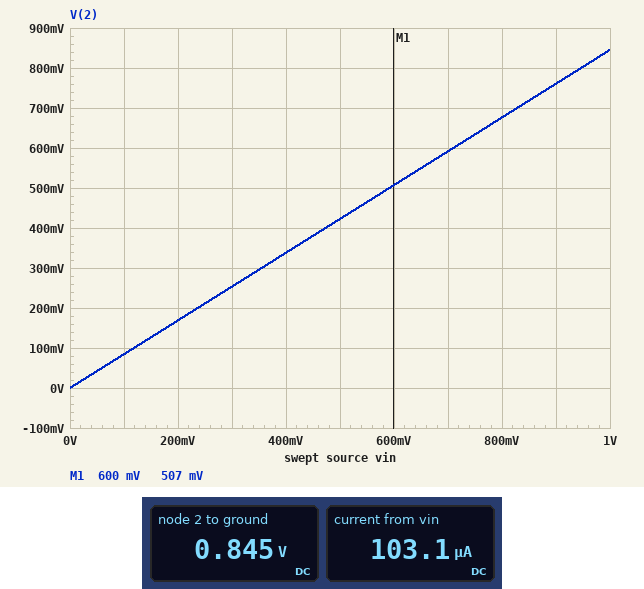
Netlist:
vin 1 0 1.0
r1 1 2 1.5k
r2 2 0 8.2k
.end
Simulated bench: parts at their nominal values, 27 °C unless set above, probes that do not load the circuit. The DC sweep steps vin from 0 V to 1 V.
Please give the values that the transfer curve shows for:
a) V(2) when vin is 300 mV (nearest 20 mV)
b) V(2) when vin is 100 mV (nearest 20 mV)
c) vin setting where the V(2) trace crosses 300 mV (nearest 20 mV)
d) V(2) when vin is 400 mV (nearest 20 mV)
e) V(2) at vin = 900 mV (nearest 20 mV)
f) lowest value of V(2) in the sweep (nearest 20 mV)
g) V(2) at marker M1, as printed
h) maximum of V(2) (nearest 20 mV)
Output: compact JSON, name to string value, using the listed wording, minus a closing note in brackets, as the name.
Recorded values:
{"V(2) when vin is 300 mV": "260 mV", "V(2) when vin is 100 mV": "80 mV", "vin setting where the V(2) trace crosses 300 mV": "360 mV", "V(2) when vin is 400 mV": "340 mV", "V(2) at vin = 900 mV": "760 mV", "lowest value of V(2) in the sweep": "0 V", "V(2) at marker M1, as printed": "507 mV", "maximum of V(2)": "840 mV"}
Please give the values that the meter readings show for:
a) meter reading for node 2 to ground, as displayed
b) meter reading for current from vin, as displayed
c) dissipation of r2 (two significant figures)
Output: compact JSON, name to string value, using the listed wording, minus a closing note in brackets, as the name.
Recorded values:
{"meter reading for node 2 to ground, as displayed": "0.845 V", "meter reading for current from vin, as displayed": "103.1 µA", "dissipation of r2": "87 µW"}
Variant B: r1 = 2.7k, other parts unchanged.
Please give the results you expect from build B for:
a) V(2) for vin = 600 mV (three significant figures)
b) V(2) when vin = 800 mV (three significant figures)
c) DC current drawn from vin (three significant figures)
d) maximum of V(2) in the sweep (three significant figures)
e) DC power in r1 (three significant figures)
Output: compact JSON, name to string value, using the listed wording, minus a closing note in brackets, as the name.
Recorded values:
{"V(2) for vin = 600 mV": "451 mV", "V(2) when vin = 800 mV": "602 mV", "DC current drawn from vin": "91.7 µA", "maximum of V(2) in the sweep": "752 mV", "DC power in r1": "22.7 µW"}
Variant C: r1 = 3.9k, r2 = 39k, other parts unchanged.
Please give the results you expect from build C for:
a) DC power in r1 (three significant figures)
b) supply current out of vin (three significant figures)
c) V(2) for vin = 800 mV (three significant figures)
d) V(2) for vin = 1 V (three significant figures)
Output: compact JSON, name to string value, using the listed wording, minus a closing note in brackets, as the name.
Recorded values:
{"DC power in r1": "2.12 µW", "supply current out of vin": "23.3 µA", "V(2) for vin = 800 mV": "727 mV", "V(2) for vin = 1 V": "909 mV"}
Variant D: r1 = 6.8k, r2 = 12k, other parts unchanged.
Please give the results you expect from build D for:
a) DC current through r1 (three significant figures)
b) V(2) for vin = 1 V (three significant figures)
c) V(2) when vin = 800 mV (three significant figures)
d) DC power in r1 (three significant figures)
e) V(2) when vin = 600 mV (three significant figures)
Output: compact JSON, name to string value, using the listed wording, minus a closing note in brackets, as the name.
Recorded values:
{"DC current through r1": "53.2 µA", "V(2) for vin = 1 V": "638 mV", "V(2) when vin = 800 mV": "511 mV", "DC power in r1": "19.2 µW", "V(2) when vin = 600 mV": "383 mV"}
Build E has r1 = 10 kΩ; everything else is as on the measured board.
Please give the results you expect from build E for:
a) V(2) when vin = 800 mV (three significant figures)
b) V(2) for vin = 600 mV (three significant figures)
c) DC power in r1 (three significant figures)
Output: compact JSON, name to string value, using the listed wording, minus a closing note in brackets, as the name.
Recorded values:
{"V(2) when vin = 800 mV": "360 mV", "V(2) for vin = 600 mV": "270 mV", "DC power in r1": "30.2 µW"}
